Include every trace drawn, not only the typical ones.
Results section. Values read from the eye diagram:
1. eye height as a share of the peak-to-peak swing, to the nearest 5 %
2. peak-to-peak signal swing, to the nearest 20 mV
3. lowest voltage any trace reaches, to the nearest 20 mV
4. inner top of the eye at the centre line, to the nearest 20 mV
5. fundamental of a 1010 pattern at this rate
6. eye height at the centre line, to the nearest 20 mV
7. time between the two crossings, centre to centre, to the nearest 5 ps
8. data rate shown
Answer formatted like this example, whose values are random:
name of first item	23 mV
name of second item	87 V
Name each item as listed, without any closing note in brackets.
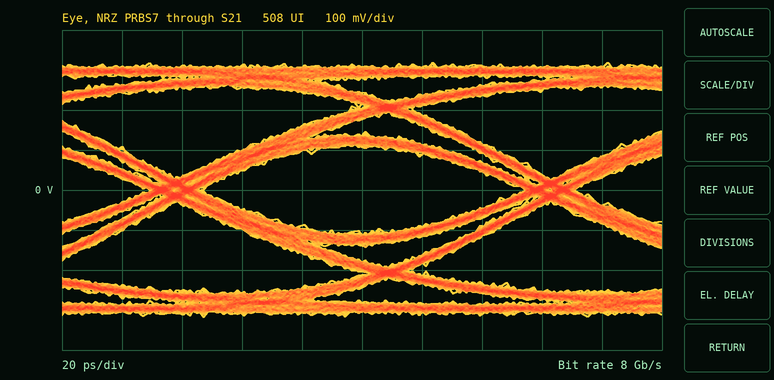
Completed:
eye height as a share of the peak-to-peak swing, to the nearest 5 %	35 %
peak-to-peak signal swing, to the nearest 20 mV	640 mV
lowest voltage any trace reaches, to the nearest 20 mV	-320 mV
inner top of the eye at the centre line, to the nearest 20 mV	100 mV
fundamental of a 1010 pattern at this rate	4 GHz
eye height at the centre line, to the nearest 20 mV	220 mV
time between the two crossings, centre to centre, to the nearest 5 ps	125 ps
data rate shown	8 Gb/s
